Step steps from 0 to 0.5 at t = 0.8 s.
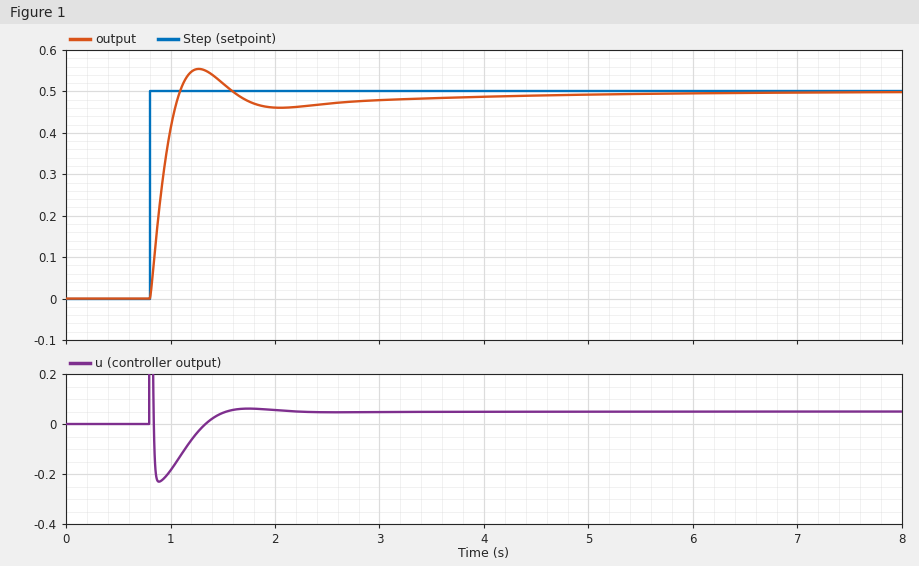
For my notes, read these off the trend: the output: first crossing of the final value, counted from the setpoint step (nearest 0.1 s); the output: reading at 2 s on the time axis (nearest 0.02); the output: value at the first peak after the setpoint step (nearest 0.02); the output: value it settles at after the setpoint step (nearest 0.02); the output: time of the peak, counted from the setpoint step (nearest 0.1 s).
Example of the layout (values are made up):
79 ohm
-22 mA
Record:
0.3 s
0.46
0.56
0.50
0.5 s
